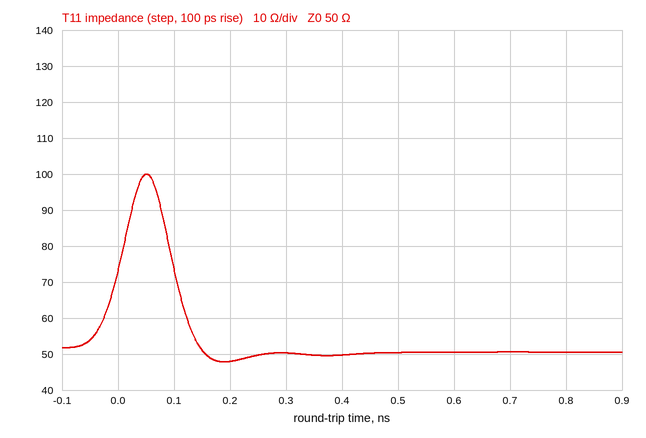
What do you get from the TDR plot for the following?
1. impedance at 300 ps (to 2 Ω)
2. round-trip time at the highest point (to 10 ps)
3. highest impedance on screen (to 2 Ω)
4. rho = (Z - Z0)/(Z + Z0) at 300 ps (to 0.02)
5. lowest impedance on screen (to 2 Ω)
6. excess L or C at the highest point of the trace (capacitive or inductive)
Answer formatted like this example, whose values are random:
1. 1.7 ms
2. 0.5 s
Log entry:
1. 50 Ω
2. 50 ps
3. 100 Ω
4. 0.00
5. 48 Ω
6. inductive
